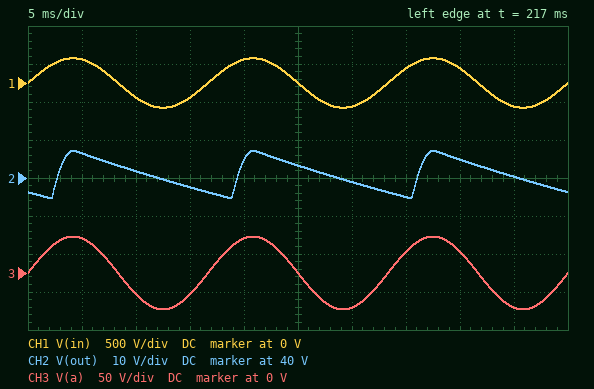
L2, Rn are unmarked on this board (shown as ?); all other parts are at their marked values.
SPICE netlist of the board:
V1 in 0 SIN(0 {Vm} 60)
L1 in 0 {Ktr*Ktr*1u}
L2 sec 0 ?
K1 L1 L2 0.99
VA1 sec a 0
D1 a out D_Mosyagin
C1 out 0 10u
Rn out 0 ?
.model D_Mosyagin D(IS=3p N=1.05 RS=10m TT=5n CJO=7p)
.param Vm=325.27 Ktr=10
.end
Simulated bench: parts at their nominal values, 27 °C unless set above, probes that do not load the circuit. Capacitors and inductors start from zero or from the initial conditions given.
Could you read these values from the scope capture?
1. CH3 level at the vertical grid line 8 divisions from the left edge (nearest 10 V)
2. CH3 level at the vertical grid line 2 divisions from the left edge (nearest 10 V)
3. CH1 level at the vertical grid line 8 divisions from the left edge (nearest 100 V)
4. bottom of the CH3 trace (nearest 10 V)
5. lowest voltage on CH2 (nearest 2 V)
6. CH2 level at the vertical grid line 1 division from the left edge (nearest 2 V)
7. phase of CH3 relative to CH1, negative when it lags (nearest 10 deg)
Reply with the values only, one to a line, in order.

30 V
-30 V
200 V
-50 V
34 V
46 V
0 deg
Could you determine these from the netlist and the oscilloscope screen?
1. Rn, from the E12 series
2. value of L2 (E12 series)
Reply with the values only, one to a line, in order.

4.7 kΩ
2.2 µH
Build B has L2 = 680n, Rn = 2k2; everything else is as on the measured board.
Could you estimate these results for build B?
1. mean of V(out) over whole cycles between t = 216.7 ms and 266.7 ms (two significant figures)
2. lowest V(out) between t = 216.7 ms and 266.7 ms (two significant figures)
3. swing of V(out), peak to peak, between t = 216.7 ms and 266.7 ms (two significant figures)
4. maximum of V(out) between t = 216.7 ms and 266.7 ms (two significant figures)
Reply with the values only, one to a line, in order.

20 V
14 V
12 V
26 V
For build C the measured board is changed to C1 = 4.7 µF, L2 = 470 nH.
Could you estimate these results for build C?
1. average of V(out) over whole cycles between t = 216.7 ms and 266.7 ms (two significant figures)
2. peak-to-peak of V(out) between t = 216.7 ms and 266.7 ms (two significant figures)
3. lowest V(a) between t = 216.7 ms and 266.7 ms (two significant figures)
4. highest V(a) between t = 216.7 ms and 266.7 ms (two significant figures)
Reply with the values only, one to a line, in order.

16 V
10 V
-22 V
22 V
